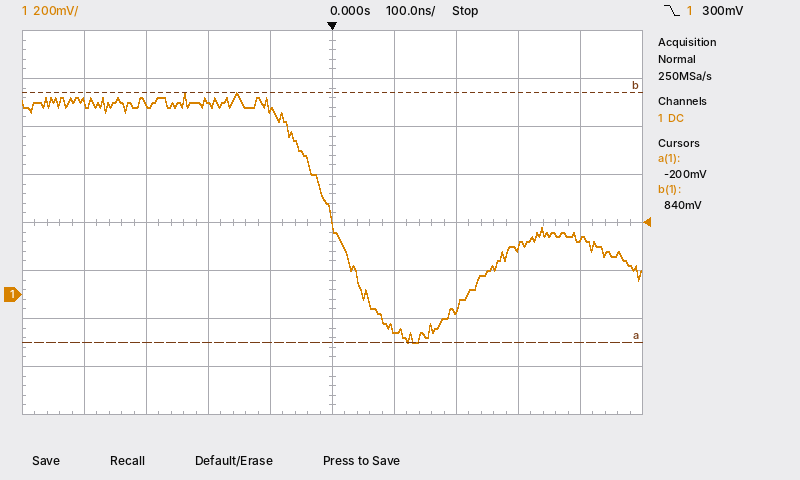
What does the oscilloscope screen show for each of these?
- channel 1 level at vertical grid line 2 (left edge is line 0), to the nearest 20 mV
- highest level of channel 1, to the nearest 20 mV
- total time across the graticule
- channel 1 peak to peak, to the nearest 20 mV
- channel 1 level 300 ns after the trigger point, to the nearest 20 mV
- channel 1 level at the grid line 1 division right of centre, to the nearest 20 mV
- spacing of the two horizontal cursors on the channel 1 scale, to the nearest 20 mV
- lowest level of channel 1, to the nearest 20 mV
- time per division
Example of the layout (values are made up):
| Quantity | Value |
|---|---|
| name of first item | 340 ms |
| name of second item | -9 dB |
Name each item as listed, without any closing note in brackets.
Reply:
| Quantity | Value |
|---|---|
| channel 1 level at vertical grid line 2 (left edge is line 0), to the nearest 20 mV | 800 mV |
| highest level of channel 1, to the nearest 20 mV | 840 mV |
| total time across the graticule | 1 µs |
| channel 1 peak to peak, to the nearest 20 mV | 1.04 V |
| channel 1 level 300 ns after the trigger point, to the nearest 20 mV | 200 mV |
| channel 1 level at the grid line 1 division right of centre, to the nearest 20 mV | -140 mV |
| spacing of the two horizontal cursors on the channel 1 scale, to the nearest 20 mV | 1.04 V |
| lowest level of channel 1, to the nearest 20 mV | -200 mV |
| time per division | 100 ns |
